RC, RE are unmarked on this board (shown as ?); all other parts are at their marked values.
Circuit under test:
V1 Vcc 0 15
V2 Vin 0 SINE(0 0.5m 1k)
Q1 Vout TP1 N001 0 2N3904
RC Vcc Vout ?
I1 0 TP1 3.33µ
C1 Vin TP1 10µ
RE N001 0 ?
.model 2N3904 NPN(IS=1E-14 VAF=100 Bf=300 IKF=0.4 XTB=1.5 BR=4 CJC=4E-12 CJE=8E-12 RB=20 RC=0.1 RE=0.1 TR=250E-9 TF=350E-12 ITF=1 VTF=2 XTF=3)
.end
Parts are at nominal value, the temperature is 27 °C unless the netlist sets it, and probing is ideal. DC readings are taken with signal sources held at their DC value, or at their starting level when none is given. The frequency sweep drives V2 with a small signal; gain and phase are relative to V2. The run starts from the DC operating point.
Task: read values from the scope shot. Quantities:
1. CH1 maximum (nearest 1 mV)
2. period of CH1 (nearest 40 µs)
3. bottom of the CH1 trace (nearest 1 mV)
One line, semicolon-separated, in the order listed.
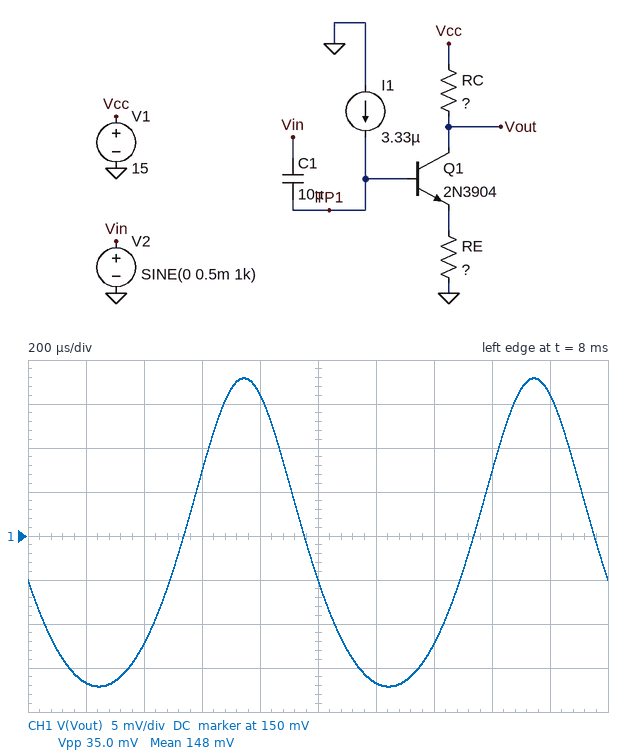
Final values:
168 mV; 1.00 ms; 133 mV
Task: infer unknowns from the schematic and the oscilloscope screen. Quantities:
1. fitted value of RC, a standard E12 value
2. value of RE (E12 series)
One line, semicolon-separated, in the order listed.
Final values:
33 kΩ; 82 Ω
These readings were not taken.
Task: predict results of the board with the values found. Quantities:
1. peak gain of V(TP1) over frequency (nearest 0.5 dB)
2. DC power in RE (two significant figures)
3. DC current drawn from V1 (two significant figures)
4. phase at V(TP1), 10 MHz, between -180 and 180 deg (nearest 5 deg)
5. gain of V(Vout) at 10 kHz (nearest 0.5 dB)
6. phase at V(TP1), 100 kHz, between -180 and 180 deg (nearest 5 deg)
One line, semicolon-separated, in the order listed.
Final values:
0 dB; 17 µW; 450 µA; 0 deg; 30.0 dB; 0 deg
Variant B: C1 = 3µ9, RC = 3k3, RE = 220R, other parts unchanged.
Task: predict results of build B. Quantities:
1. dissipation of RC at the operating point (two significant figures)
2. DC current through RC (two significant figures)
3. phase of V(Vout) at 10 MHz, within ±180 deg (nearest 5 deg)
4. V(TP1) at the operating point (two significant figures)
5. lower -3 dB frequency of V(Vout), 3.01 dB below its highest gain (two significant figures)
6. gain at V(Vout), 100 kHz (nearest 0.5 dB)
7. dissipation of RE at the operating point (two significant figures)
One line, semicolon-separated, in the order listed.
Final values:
4.0 mW; 1.1 mA; 155 deg; 900 mV; 520 mHz; 22.5 dB; 270 µW
